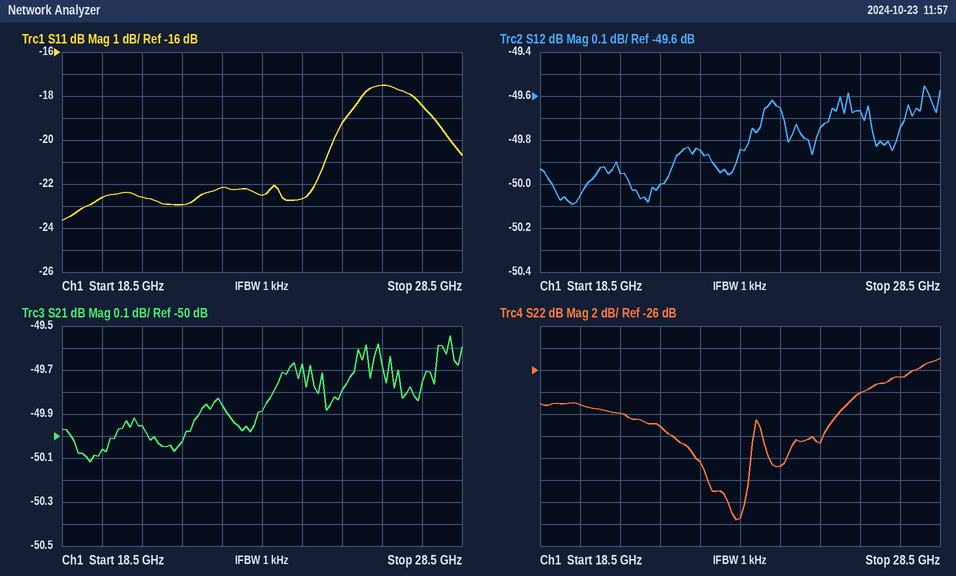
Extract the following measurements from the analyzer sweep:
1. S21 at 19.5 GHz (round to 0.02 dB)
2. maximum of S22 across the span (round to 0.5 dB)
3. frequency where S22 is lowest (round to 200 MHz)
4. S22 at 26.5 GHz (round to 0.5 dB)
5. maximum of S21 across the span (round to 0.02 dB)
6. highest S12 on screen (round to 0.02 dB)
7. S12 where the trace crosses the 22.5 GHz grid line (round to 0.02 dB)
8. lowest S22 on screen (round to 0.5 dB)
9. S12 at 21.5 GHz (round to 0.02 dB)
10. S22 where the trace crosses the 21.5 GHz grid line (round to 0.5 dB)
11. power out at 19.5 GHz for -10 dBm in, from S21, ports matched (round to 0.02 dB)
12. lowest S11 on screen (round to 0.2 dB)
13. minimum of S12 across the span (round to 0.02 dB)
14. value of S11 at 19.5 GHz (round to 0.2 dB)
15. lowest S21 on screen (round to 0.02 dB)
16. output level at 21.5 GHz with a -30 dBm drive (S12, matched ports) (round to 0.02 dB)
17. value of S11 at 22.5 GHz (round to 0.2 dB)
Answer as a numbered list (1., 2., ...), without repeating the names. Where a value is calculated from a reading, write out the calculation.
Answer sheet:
1. -50.06 dB
2. -25.0 dB
3. 23.4 GHz
4. -28.0 dB
5. -49.54 dB
6. -49.56 dB
7. -49.84 dB
8. -39.5 dB
9. -50.00 dB
10. -31.0 dB
11. -10 dBm + (-50.06 dB) = -60.06 dBm
12. -23.6 dB
13. -50.10 dB
14. -22.6 dB
15. -50.12 dB
16. -30 dBm + (-50.00 dB) = -80.00 dBm
17. -22.2 dB
